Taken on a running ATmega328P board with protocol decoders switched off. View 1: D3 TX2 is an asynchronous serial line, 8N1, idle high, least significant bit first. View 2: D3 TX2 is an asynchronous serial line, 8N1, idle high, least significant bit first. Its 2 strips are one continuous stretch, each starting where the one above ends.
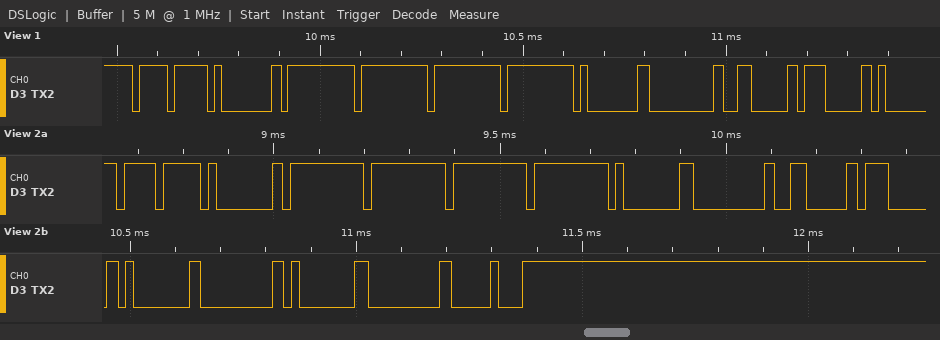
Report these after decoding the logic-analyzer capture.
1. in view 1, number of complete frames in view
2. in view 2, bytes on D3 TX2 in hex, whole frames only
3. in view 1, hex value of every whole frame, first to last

10
EF 01 FF FF FF FF 01 00 06 07 01 00 01 00 10
0xEF 0x01 0xFF 0xFF 0xFF 0xFF 0x01 0x00 0x06 0x07
